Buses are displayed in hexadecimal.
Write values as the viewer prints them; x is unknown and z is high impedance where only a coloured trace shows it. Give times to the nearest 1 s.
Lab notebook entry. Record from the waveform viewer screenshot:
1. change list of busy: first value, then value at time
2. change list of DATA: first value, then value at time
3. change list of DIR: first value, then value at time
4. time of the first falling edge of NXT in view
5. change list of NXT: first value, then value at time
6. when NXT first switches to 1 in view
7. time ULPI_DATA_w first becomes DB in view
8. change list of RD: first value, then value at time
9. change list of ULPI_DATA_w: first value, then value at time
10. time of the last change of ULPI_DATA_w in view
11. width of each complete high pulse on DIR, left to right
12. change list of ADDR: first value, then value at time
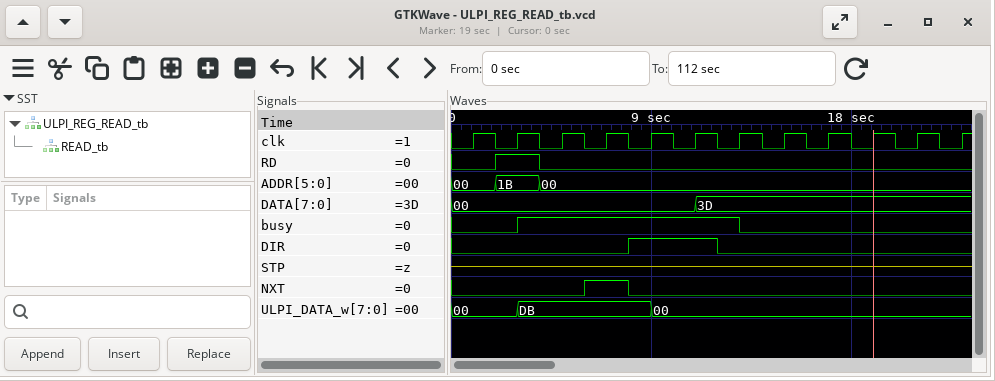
0, 1 at 3 s, 0 at 13 s
00, 3D at 11 s
0, 1 at 8 s, 0 at 12 s
8 s
0, 1 at 6 s, 0 at 8 s
6 s
3 s
0, 1 at 2 s, 0 at 4 s
00, DB at 3 s, 00 at 9 s
9 s
4 s
00, 1B at 2 s, 00 at 4 s
